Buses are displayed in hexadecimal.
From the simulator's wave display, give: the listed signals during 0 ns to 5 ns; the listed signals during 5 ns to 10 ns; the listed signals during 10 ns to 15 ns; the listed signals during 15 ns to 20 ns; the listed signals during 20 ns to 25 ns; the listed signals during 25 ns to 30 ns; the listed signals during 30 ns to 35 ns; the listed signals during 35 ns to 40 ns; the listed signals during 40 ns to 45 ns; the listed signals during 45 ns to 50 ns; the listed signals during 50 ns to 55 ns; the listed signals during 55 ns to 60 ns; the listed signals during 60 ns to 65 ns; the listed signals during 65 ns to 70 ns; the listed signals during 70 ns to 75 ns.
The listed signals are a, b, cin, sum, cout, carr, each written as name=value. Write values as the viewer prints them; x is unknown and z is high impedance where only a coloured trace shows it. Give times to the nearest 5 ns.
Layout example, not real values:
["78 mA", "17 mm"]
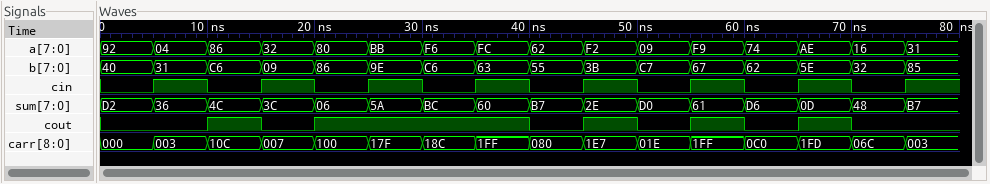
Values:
["a=92, b=40, cin=0, sum=D2, cout=0, carr=000", "a=04, b=31, cin=1, sum=36, cout=0, carr=003", "a=86, b=C6, cin=0, sum=4C, cout=1, carr=10C", "a=32, b=09, cin=1, sum=3C, cout=0, carr=007", "a=80, b=86, cin=0, sum=06, cout=1, carr=100", "a=BB, b=9E, cin=1, sum=5A, cout=1, carr=17F", "a=F6, b=C6, cin=0, sum=BC, cout=1, carr=18C", "a=FC, b=63, cin=1, sum=60, cout=1, carr=1FF", "a=62, b=55, cin=0, sum=B7, cout=0, carr=080", "a=F2, b=3B, cin=1, sum=2E, cout=1, carr=1E7", "a=09, b=C7, cin=0, sum=D0, cout=0, carr=01E", "a=F9, b=67, cin=1, sum=61, cout=1, carr=1FF", "a=74, b=62, cin=0, sum=D6, cout=0, carr=0C0", "a=AE, b=5E, cin=1, sum=0D, cout=1, carr=1FD", "a=16, b=32, cin=0, sum=48, cout=0, carr=06C"]
